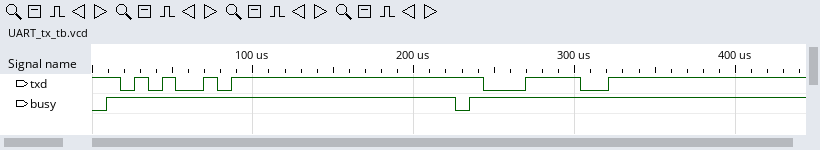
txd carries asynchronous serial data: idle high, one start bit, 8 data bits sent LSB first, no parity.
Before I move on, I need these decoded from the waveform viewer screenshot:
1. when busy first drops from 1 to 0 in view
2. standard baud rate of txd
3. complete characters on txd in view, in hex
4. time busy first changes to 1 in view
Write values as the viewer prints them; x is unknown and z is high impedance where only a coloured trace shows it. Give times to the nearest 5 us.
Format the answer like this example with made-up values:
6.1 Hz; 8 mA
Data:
225 us; 115200 baud; A5, 3C; 10 us
